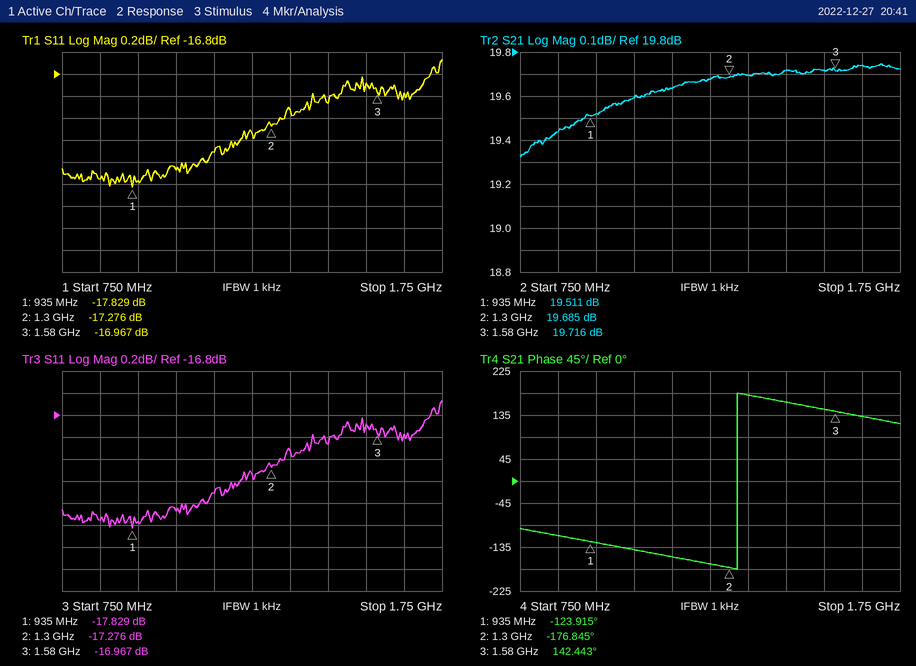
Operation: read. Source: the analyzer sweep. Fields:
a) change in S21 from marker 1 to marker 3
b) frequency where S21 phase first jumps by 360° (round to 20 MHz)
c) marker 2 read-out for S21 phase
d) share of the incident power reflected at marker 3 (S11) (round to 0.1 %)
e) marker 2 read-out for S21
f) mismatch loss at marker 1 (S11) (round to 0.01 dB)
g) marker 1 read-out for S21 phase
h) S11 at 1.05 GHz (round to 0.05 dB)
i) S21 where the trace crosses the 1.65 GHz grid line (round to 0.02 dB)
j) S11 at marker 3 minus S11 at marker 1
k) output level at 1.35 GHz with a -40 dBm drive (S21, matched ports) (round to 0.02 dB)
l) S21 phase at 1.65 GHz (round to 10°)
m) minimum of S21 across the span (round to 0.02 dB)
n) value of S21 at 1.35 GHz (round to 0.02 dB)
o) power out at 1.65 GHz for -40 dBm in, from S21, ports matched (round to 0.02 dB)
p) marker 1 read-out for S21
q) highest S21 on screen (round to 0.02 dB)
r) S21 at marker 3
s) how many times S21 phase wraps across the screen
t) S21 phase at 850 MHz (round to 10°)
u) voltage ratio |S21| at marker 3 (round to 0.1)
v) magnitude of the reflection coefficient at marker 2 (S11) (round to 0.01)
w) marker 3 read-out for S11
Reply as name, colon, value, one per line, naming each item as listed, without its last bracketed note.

change in S21 from marker 1 to marker 3: 0.205 dB
frequency where S21 phase first jumps by 360°: 1.32 GHz
marker 2 read-out for S21 phase: -176.845°
share of the incident power reflected at marker 3 (S11): 2.0 %
marker 2 read-out for S21: 19.685 dB
mismatch loss at marker 1 (S11): 0.07 dB
marker 1 read-out for S21 phase: -123.915°
S11 at 1.05 GHz: -17.65 dB
S21 where the trace crosses the 1.65 GHz grid line: 19.74 dB
S11 at marker 3 minus S11 at marker 1: 0.862 dB
output level at 1.35 GHz with a -40 dBm drive (S21, matched ports): -20.30 dBm
S21 phase at 1.65 GHz: 130°
minimum of S21 across the span: 19.32 dB
value of S21 at 1.35 GHz: 19.70 dB
power out at 1.65 GHz for -40 dBm in, from S21, ports matched: -20.26 dBm
marker 1 read-out for S21: 19.511 dB
highest S21 on screen: 19.74 dB
S21 at marker 3: 19.716 dB
how many times S21 phase wraps across the screen: 1
S21 phase at 850 MHz: -110°
voltage ratio |S21| at marker 3: 9.7
magnitude of the reflection coefficient at marker 2 (S11): 0.14
marker 3 read-out for S11: -16.967 dB
